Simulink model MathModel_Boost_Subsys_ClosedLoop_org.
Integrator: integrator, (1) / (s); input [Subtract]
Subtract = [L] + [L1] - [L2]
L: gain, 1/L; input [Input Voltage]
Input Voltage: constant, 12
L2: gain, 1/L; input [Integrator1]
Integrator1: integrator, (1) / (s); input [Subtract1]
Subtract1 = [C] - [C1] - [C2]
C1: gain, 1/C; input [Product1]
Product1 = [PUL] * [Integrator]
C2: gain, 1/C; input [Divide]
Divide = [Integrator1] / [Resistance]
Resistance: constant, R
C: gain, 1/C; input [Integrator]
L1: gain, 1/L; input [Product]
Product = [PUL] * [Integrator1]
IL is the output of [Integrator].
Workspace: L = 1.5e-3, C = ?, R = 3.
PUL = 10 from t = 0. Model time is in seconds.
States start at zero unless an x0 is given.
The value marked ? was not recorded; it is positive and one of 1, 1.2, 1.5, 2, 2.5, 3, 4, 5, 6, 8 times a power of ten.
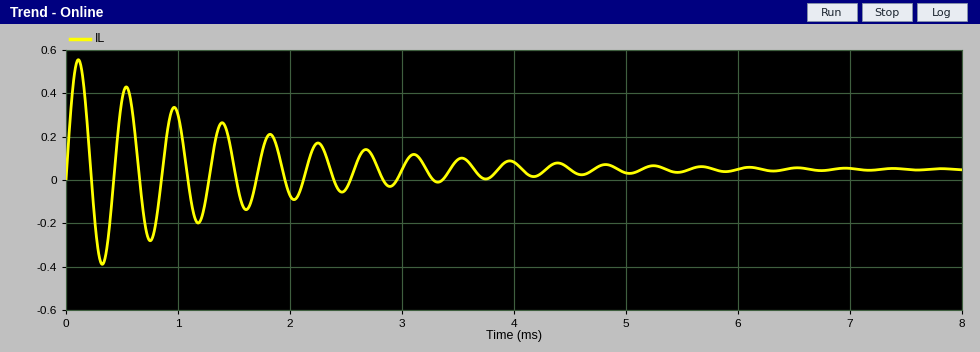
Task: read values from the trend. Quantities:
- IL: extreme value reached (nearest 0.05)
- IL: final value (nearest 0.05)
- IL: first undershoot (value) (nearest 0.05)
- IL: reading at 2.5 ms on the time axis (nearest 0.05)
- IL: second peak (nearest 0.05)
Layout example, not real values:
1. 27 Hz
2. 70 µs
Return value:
1. 0.55
2. 0.05
3. -0.40
4. -0.05
5. 0.45
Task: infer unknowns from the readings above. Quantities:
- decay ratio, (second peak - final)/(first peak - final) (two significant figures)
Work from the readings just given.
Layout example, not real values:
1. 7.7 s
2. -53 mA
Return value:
1. 0.80
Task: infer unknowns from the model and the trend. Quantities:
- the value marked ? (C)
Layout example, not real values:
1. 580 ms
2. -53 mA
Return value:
1. 0.00025
